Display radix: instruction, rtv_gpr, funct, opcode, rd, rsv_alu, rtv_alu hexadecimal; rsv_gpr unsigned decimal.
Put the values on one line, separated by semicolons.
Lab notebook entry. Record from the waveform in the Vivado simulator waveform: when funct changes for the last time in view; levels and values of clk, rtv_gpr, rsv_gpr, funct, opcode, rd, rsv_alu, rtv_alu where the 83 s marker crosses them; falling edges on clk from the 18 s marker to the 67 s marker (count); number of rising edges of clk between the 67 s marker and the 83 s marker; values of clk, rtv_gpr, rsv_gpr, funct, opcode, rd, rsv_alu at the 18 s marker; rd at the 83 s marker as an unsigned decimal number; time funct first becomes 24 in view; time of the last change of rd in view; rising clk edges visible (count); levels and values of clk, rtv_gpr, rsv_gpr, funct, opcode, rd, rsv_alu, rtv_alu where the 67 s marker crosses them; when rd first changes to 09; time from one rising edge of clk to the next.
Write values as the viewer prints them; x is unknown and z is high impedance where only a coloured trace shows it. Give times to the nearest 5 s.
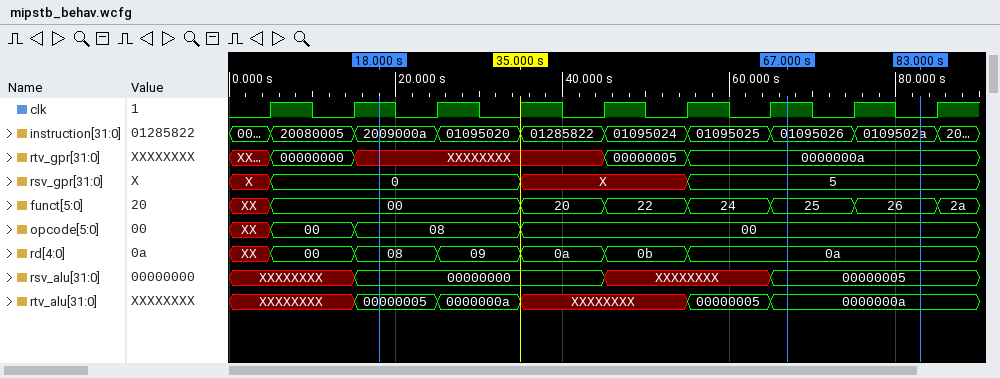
85 s; clk=0, rtv_gpr=0000000a, rsv_gpr=5, funct=26, opcode=00, rd=0a, rsv_alu=00000005, rtv_alu=0000000a; 5; 1; clk=1, rtv_gpr=XXXXXXXX, rsv_gpr=0, funct=00, opcode=08, rd=08, rsv_alu=00000000; 10; 55 s; 55 s; 9; clk=1, rtv_gpr=0000000a, rsv_gpr=5, funct=25, opcode=00, rd=0a, rsv_alu=00000005, rtv_alu=0000000a; 25 s; 10 s
